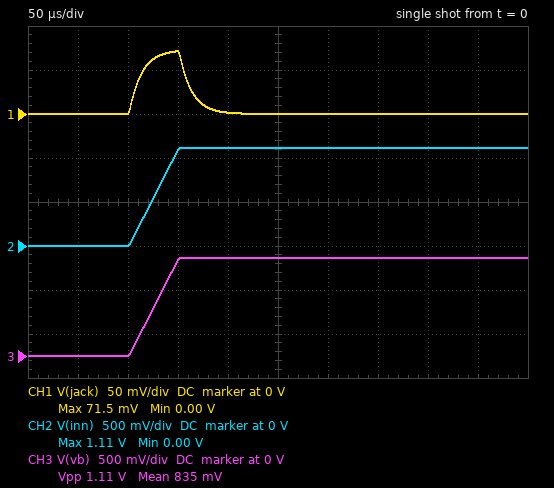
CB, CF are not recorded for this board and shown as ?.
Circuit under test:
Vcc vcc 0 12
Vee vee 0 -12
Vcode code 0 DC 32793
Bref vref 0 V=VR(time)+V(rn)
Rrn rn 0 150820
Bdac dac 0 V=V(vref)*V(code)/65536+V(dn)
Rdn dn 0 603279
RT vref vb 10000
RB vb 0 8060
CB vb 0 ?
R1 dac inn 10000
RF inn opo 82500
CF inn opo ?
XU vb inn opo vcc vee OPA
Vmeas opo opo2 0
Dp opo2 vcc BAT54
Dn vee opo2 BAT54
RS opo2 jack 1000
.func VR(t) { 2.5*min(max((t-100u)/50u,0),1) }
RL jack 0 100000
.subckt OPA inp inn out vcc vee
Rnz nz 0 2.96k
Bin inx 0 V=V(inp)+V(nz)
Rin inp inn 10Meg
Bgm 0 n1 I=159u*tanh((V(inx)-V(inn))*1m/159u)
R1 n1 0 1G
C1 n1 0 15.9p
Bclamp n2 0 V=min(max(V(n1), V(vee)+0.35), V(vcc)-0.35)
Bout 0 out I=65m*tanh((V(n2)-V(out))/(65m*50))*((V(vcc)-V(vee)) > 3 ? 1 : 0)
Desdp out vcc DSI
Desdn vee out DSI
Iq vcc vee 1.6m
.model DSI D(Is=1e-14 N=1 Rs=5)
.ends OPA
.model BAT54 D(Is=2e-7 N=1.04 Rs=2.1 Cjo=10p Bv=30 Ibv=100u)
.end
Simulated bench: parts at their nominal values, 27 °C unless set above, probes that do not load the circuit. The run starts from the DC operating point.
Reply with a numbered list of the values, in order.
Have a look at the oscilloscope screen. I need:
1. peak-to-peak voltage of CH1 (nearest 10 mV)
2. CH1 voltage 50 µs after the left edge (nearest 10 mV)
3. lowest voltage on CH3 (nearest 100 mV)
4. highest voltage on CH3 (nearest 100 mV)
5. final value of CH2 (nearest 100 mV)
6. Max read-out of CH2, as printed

1. 70 mV
2. 0 V
3. 0 V
4. 1.1 V
5. 1.1 V
6. 1.11 V
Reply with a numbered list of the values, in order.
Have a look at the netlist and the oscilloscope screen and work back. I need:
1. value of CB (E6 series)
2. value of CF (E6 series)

1. 220 pF
2. 150 pF
